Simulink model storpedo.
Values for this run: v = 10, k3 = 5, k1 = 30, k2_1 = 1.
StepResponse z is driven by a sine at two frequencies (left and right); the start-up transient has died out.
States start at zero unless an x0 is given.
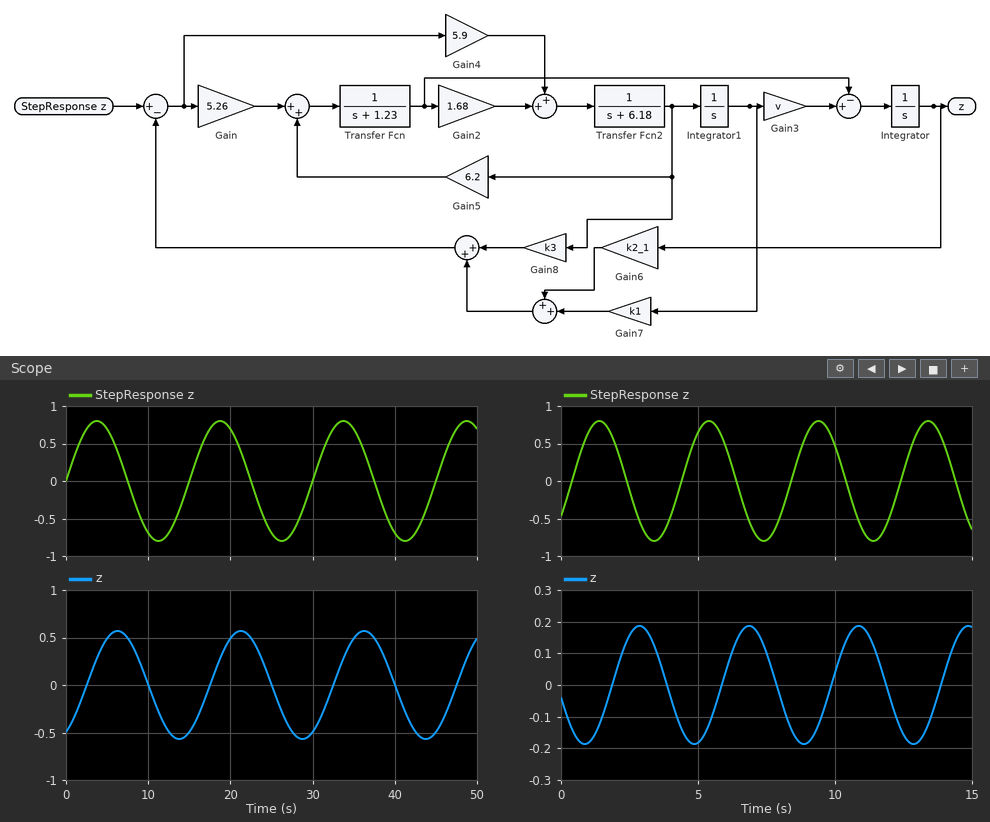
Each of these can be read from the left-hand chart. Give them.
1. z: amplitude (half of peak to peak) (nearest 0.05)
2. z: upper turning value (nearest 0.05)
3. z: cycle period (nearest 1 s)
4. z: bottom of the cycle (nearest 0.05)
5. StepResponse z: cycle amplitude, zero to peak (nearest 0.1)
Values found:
0.55
0.55
15 s
-0.55
0.8
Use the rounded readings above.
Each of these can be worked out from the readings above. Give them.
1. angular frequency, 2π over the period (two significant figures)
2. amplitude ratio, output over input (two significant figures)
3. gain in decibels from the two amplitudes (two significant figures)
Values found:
0.42 rad/s
0.69
-3.3 dB
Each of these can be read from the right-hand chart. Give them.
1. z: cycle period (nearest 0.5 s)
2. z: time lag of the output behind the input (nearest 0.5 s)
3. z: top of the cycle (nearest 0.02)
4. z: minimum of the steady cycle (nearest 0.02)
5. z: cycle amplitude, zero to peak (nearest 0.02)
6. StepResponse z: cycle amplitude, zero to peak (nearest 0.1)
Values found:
4.0 s
1.5 s
0.18
-0.18
0.18
0.8
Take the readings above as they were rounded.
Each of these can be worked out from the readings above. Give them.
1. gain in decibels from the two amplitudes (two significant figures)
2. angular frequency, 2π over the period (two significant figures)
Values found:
-13 dB
1.6 rad/s
